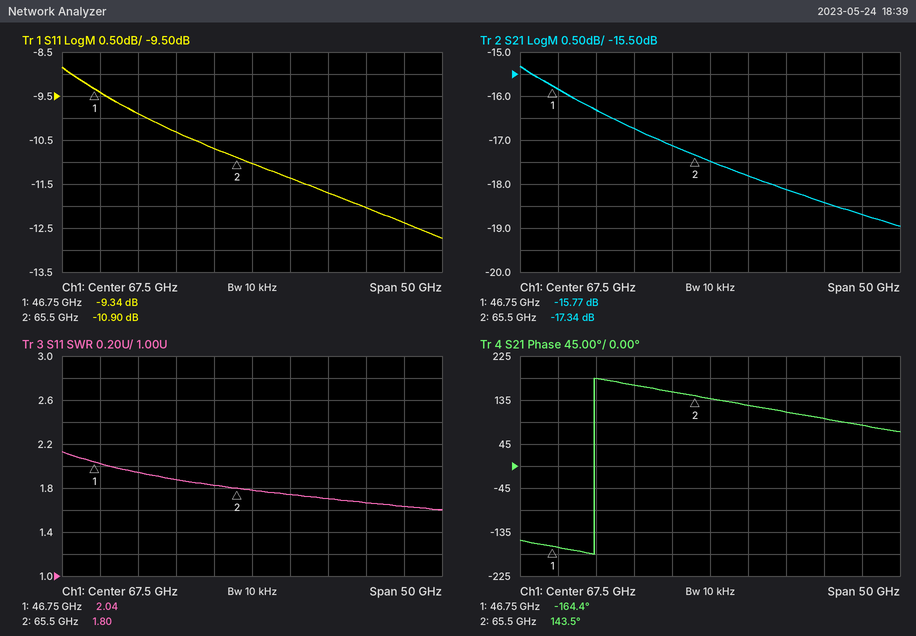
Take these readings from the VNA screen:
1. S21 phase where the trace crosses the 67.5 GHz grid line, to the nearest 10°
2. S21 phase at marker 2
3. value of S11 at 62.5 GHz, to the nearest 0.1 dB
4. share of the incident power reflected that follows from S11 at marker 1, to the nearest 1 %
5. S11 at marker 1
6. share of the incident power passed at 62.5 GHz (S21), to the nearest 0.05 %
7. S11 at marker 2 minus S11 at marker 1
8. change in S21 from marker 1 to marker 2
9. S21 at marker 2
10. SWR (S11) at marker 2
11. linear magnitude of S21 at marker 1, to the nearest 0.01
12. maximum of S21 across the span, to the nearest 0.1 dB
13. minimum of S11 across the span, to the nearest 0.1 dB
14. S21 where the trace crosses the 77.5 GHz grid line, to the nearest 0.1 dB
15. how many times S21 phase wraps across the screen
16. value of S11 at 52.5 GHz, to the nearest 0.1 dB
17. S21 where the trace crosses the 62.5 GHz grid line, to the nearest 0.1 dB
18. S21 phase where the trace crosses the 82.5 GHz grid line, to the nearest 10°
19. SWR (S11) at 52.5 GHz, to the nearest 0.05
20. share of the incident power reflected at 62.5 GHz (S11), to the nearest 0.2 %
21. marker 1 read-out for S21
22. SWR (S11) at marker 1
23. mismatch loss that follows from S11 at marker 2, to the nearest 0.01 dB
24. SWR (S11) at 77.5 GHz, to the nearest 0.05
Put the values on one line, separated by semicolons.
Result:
140°; 143.5°; -10.7 dB; 12 %; -9.34 dB; 1.95 %; -1.56 dB; -1.57 dB; -17.34 dB; 1.80; 0.16; -15.3 dB; -12.7 dB; -18.1 dB; 1; -9.9 dB; -17.1 dB; 100°; 1.95; 8.6 %; -15.77 dB; 2.04; 0.37 dB; 1.70
